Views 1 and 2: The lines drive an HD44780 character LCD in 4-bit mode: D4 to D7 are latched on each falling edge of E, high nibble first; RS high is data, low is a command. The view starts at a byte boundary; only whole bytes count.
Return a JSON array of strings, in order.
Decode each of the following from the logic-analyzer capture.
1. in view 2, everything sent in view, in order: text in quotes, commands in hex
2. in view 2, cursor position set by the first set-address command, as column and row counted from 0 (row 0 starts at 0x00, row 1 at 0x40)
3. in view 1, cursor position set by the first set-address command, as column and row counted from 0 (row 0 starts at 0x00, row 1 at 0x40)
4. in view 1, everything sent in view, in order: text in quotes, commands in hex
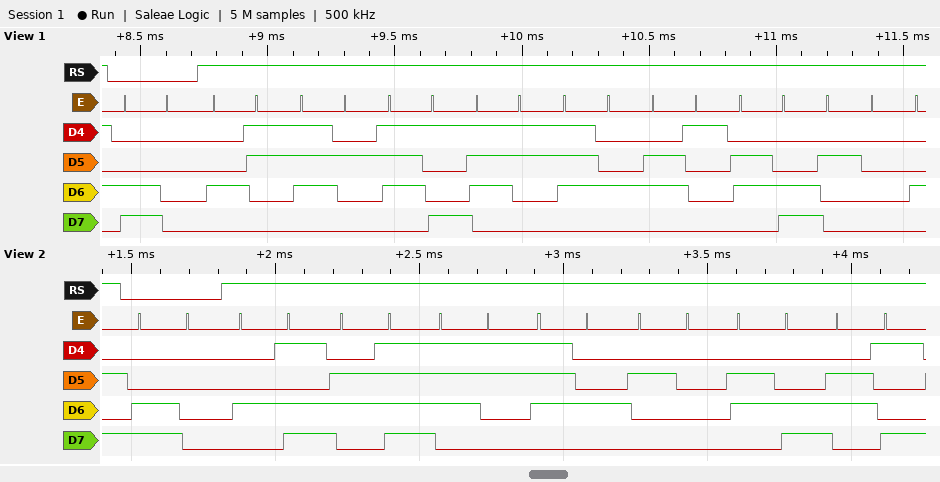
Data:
["0xC0 \"Most li\"", "column 0, row 1", "column 0, row 1", "0xC0 \"Crystal \""]
